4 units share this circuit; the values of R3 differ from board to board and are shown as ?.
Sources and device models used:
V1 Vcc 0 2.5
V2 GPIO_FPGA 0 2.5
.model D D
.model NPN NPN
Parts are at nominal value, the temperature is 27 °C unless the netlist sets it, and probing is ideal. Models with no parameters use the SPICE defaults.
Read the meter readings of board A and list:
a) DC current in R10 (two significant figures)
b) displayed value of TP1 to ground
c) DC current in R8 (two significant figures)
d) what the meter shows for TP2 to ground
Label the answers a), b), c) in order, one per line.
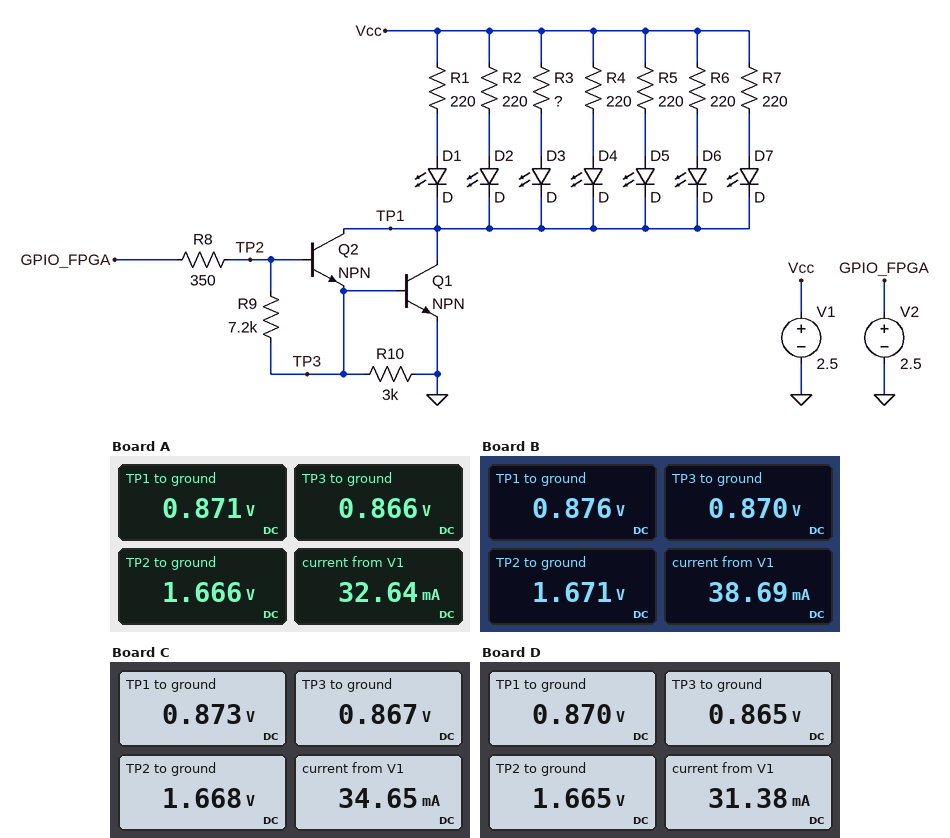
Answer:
a) 290 µA
b) 0.871 V
c) 2.4 mA
d) 1.666 V
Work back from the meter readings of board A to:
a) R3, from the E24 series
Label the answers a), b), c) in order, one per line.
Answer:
a) 130 Ω
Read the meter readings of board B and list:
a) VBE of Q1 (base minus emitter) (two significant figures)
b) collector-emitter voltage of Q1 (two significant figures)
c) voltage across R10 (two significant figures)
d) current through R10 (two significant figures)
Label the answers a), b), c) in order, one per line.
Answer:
a) 870 mV
b) 880 mV
c) 870 mV
d) 290 µA
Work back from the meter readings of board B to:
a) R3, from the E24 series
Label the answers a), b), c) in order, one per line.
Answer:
a) 68 Ω
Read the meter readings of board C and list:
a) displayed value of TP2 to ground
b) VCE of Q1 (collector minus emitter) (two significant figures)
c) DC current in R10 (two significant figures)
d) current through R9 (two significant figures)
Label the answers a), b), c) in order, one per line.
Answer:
a) 1.668 V
b) 870 mV
c) 290 µA
d) 110 µA
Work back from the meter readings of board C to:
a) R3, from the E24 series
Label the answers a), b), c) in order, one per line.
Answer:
a) 100 Ω
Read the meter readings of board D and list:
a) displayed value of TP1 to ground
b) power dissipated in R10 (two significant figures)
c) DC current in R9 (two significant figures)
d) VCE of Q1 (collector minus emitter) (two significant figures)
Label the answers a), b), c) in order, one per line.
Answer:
a) 0.870 V
b) 250 µW
c) 110 µA
d) 870 mV
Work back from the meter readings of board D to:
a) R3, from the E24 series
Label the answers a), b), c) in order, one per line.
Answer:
a) 160 Ω
